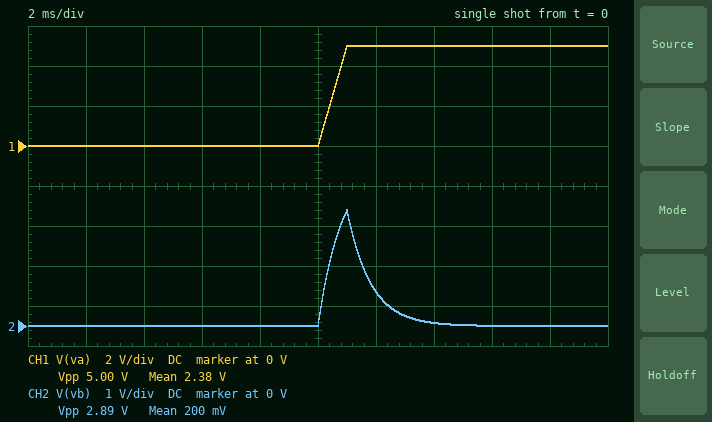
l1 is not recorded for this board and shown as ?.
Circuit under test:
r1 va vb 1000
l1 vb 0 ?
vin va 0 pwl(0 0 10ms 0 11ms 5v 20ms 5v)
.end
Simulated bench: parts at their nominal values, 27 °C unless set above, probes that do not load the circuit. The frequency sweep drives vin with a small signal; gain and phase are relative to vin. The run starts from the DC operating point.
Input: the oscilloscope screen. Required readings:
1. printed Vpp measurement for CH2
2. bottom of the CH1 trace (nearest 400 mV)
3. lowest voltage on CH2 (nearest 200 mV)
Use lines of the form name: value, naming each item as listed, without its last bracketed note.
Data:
printed Vpp measurement for CH2: 2.89 V
bottom of the CH1 trace: 0 V
lowest voltage on CH2: 0 V
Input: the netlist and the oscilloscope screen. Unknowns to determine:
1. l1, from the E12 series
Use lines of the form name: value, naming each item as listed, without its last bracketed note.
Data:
l1, from the E12 series: 820 mH
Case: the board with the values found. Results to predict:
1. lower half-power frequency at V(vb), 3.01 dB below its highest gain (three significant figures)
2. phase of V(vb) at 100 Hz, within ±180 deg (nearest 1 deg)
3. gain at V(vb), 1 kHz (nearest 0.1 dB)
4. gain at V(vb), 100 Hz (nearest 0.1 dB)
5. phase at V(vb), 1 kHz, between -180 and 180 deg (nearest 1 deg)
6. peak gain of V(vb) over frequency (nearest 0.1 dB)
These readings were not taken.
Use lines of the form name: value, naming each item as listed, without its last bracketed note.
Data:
lower half-power frequency at V(vb), 3.01 dB below its highest gain: 194 Hz
phase of V(vb) at 100 Hz, within ±180 deg: 63 deg
gain at V(vb), 1 kHz: -0.2 dB
gain at V(vb), 100 Hz: -6.8 dB
phase at V(vb), 1 kHz, between -180 and 180 deg: 11 deg
peak gain of V(vb) over frequency: 0 dB
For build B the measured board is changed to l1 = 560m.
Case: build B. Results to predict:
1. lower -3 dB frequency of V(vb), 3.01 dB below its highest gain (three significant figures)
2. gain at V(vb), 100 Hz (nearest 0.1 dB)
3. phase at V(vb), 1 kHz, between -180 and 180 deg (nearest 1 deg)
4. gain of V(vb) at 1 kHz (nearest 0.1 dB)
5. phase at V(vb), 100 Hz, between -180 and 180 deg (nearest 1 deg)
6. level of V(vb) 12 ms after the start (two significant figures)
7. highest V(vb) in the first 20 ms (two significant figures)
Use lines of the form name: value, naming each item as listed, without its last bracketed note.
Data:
lower -3 dB frequency of V(vb), 3.01 dB below its highest gain: 284 Hz
gain at V(vb), 100 Hz: -9.6 dB
phase at V(vb), 1 kHz, between -180 and 180 deg: 16 deg
gain of V(vb) at 1 kHz: -0.3 dB
phase at V(vb), 100 Hz, between -180 and 180 deg: 71 deg
level of V(vb) 12 ms after the start: 390 mV
highest V(vb) in the first 20 ms: 2.3 V
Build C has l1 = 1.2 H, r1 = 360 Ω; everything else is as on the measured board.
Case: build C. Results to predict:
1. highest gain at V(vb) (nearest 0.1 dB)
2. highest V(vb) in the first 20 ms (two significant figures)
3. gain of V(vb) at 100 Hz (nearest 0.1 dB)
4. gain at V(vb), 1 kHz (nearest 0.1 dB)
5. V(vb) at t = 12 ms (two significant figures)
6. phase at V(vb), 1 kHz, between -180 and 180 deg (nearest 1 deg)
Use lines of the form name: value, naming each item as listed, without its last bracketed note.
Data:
highest gain at V(vb): 0 dB
highest V(vb) in the first 20 ms: 4.3 V
gain of V(vb) at 100 Hz: -0.9 dB
gain at V(vb), 1 kHz: 0 dB
V(vb) at t = 12 ms: 3.2 V
phase at V(vb), 1 kHz, between -180 and 180 deg: 3 deg
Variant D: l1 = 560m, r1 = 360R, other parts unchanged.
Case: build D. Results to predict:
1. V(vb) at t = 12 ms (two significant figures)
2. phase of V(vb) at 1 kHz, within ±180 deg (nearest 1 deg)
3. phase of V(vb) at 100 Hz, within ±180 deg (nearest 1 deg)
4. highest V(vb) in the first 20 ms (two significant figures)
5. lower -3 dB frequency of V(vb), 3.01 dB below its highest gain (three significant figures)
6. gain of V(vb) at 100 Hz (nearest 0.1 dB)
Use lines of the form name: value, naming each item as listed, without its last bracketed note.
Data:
V(vb) at t = 12 ms: 1.9 V
phase of V(vb) at 1 kHz, within ±180 deg: 6 deg
phase of V(vb) at 100 Hz, within ±180 deg: 46 deg
highest V(vb) in the first 20 ms: 3.7 V
lower -3 dB frequency of V(vb), 3.01 dB below its highest gain: 102 Hz
gain of V(vb) at 100 Hz: -3.1 dB
